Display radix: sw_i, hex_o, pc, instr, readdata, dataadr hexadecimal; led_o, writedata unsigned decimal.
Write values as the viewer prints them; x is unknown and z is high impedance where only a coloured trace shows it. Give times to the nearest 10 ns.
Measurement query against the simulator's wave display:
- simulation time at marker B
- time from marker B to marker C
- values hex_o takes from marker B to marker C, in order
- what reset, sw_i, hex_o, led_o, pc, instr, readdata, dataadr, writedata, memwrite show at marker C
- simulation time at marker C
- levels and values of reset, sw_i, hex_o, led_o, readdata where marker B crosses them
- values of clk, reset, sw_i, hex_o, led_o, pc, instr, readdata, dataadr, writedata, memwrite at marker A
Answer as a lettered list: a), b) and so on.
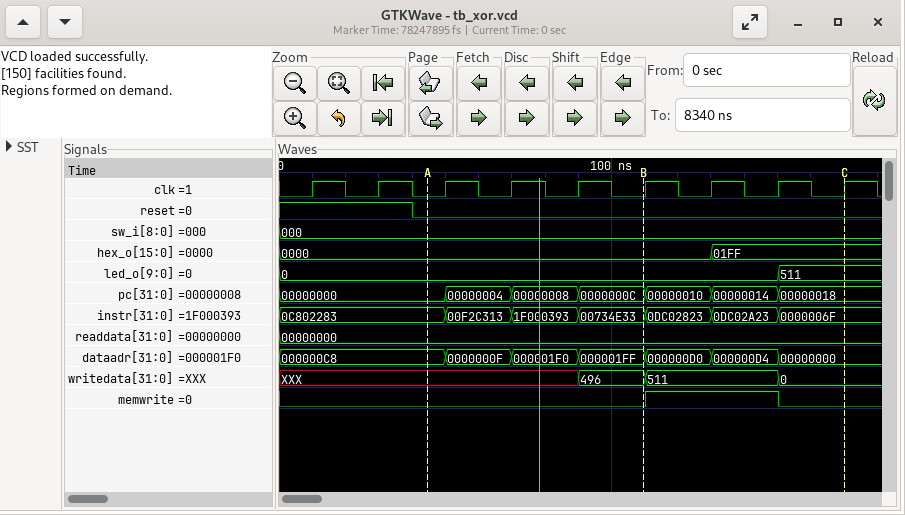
a) 110 ns
b) 60 ns
c) 0000, 01FF
d) reset=0, sw_i=000, hex_o=01FF, led_o=511, pc=00000018, instr=0000006F, readdata=00000000, dataadr=00000000, writedata=0, memwrite=0
e) 170 ns
f) reset=0, sw_i=000, hex_o=0000, led_o=0, readdata=00000000
g) clk=0, reset=0, sw_i=000, hex_o=0000, led_o=0, pc=00000000, instr=0C802283, readdata=00000000, dataadr=000000C8, writedata=XXX, memwrite=0
